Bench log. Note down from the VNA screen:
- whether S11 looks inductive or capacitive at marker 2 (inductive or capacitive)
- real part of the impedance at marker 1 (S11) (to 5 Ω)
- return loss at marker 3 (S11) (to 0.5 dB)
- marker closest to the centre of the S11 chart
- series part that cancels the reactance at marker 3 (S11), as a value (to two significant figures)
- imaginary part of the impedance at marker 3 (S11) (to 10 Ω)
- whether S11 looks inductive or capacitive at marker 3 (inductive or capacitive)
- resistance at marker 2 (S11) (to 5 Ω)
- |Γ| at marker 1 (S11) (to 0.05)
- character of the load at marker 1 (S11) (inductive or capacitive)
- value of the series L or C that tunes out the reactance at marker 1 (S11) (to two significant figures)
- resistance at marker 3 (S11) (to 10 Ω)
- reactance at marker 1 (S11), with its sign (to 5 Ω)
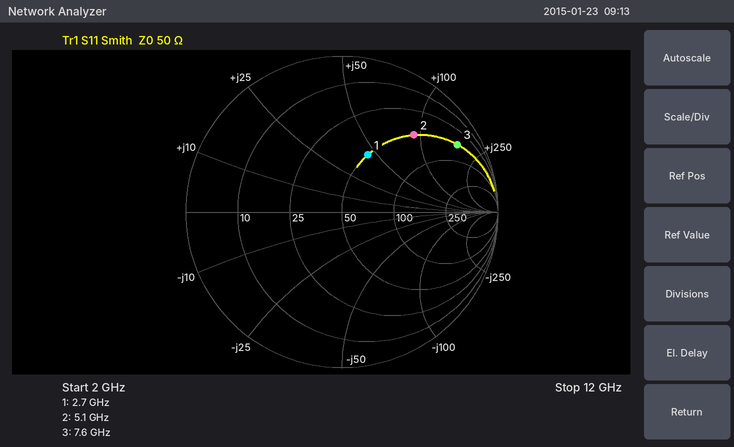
inductive
50 Ω
1.5 dB
marker 1
120 fF
+170 Ω
inductive
50 Ω
0.40
inductive
1.3 pF
50 Ω
+45 Ω
